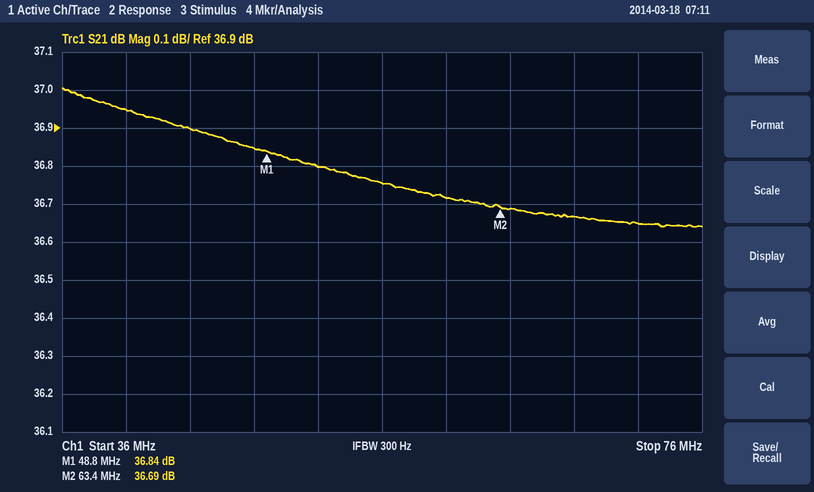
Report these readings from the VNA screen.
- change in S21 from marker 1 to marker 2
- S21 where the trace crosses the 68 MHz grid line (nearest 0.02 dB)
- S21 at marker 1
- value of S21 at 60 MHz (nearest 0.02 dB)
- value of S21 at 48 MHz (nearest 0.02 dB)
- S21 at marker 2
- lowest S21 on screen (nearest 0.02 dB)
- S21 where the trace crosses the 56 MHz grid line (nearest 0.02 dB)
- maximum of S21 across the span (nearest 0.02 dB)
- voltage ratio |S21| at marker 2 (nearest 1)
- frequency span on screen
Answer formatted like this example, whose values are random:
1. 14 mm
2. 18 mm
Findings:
1. -0.15 dB
2. 36.66 dB
3. 36.84 dB
4. 36.72 dB
5. 36.84 dB
6. 36.69 dB
7. 36.64 dB
8. 36.76 dB
9. 37.00 dB
10. 68
11. 40 MHz
